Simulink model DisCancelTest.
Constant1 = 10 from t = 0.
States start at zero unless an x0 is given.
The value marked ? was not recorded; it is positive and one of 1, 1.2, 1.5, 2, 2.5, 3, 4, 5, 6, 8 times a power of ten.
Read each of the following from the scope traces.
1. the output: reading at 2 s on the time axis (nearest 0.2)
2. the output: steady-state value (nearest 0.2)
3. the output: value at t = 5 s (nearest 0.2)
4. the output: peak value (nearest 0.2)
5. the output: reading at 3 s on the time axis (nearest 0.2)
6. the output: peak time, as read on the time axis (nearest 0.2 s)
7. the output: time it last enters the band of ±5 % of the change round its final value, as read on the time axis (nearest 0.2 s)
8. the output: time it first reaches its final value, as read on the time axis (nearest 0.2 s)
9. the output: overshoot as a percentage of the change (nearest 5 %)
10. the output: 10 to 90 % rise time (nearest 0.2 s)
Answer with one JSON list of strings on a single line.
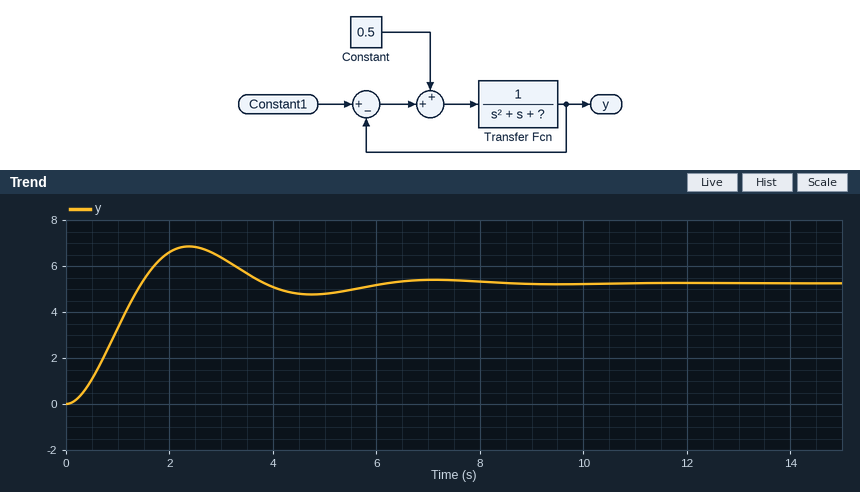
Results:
["6.6", "5.2", "4.8", "6.8", "6.4", "2.4 s", "5.6 s", "1.4 s", "30 %", "1.0 s"]
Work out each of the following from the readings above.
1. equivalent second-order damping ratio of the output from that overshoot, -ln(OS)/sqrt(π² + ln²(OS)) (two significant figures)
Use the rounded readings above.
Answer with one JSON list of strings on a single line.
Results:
["0.36"]
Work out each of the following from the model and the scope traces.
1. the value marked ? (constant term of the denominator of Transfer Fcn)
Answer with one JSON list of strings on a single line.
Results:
["1"]
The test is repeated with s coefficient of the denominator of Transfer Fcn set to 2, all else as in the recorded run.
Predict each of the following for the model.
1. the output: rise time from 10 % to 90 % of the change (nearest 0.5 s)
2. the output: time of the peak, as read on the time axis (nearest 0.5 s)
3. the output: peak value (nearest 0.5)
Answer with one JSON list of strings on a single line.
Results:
["1.5 s", "3.0 s", "5.5"]
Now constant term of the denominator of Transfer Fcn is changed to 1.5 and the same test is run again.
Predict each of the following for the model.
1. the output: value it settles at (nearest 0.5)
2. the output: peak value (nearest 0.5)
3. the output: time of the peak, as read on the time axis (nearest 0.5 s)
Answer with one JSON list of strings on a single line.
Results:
["4.0", "5.5", "2.0 s"]
